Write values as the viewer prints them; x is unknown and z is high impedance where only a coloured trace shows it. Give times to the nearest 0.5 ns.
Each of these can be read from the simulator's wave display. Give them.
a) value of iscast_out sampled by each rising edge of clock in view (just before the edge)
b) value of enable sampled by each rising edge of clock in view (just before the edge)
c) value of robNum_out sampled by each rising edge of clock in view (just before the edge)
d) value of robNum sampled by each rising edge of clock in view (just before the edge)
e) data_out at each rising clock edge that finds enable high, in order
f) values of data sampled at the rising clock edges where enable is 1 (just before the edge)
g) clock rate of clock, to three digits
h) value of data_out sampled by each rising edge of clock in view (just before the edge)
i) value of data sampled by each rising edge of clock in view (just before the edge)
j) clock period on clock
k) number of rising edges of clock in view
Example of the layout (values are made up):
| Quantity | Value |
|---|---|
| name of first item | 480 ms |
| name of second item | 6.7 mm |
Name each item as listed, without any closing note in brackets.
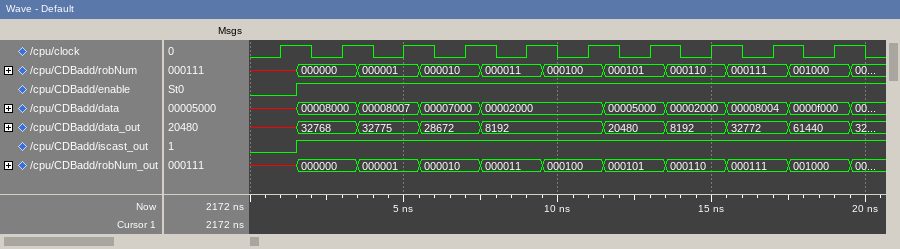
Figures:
| Quantity | Value |
|---|---|
| value of iscast_out sampled by each rising edge of clock in view | 0 1 1 1 1 1 1 1 1 1 |
| value of enable sampled by each rising edge of clock in view | 0 1 1 1 1 1 1 1 1 1 |
| value of robNum_out sampled by each rising edge of clock in view | x, 000000, 000001, 000010, 000011, 000100, 000101, 000110, 000111, 001000 |
| value of robNum sampled by each rising edge of clock in view | x, 000000, 000001, 000010, 000011, 000100, 000101, 000110, 000111, 001000 |
| data_out at each rising clock edge that finds enable high, in order | 32768, 32775, 28672, 8192, 8192, 20480, 8192, 32772, 61440 |
| values of data sampled at the rising clock edges where enable is 1 | 00008000, 00008007, 00007000, 00002000, 00002000, 00005000, 00002000, 00008004, 0000f000 |
| clock rate of clock, to three digits | 500 MHz |
| value of data_out sampled by each rising edge of clock in view | x, 32768, 32775, 28672, 8192, 8192, 20480, 8192, 32772, 61440 |
| value of data sampled by each rising edge of clock in view | x, 00008000, 00008007, 00007000, 00002000, 00002000, 00005000, 00002000, 00008004, 0000f000 |
| clock period on clock | 2 ns |
| number of rising edges of clock in view | 10 |
